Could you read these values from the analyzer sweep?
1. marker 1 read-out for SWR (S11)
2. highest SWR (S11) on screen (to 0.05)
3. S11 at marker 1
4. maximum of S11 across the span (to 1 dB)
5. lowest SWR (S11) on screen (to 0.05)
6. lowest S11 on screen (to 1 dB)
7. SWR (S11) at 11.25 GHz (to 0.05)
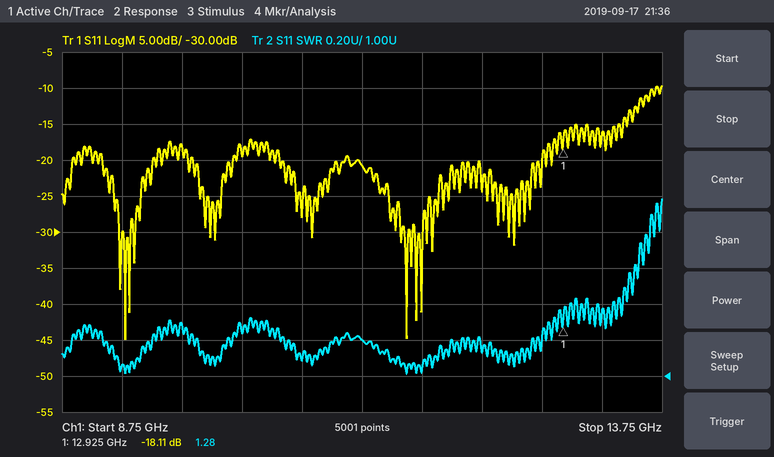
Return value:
1.28
2.00
-18.11 dB
-10 dB
1.00
-45 dB
1.20
